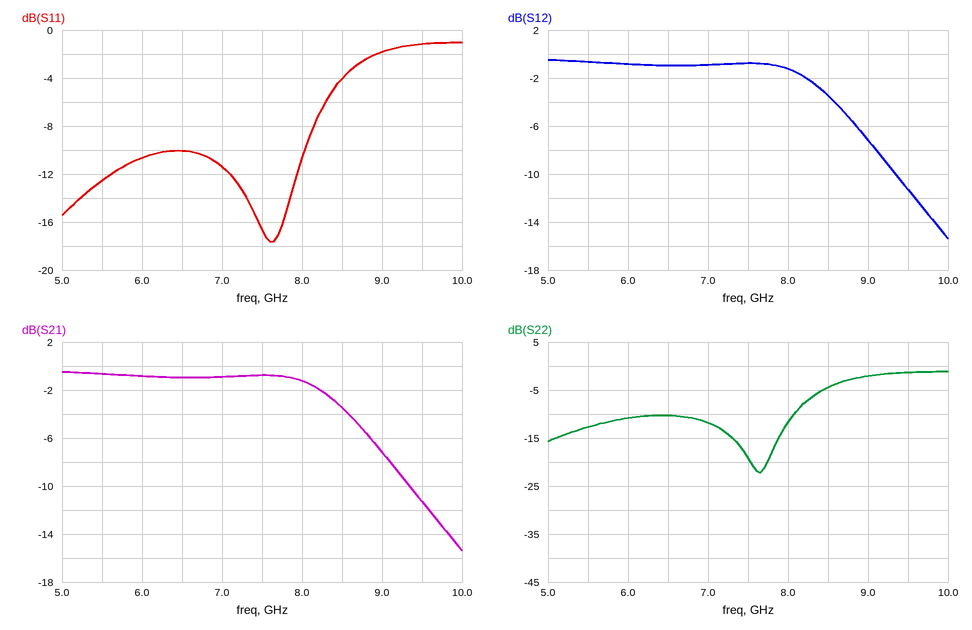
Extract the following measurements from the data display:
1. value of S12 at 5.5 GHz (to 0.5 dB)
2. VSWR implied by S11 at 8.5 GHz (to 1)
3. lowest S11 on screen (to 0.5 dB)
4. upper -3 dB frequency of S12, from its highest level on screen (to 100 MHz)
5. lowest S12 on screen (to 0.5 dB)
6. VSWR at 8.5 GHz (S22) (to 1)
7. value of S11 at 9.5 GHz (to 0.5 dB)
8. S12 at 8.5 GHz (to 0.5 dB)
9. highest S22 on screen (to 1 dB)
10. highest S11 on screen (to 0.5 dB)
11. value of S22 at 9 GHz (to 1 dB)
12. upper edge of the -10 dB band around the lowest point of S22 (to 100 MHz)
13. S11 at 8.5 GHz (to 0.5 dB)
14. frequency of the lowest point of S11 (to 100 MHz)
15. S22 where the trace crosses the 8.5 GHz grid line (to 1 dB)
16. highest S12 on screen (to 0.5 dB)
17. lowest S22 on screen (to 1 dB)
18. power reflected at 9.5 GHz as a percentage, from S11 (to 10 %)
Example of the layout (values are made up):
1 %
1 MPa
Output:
-0.5 dB
4
-17.5 dB
8.5 GHz
-15.5 dB
4
-1.0 dB
-3.5 dB
-1 dB
-1.0 dB
-2 dB
8.1 GHz
-4.0 dB
7.6 GHz
-4 dB
-0.5 dB
-22 dB
80 %
